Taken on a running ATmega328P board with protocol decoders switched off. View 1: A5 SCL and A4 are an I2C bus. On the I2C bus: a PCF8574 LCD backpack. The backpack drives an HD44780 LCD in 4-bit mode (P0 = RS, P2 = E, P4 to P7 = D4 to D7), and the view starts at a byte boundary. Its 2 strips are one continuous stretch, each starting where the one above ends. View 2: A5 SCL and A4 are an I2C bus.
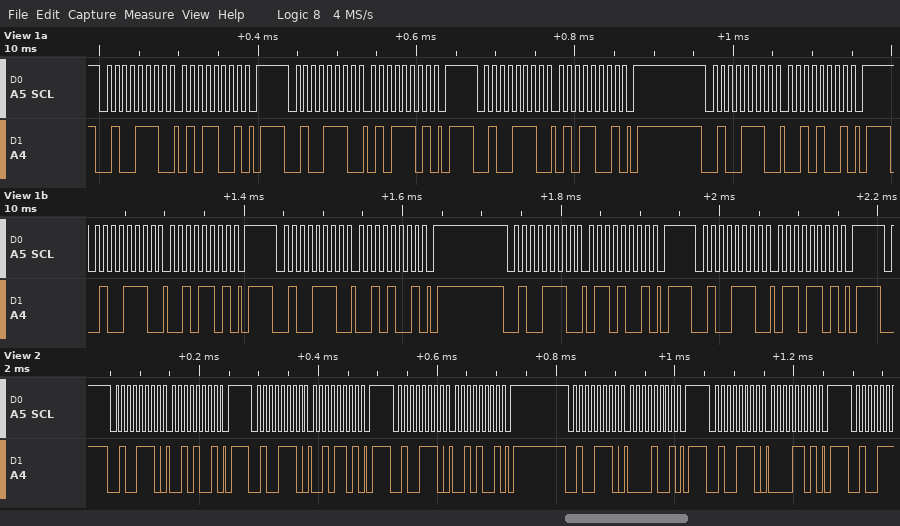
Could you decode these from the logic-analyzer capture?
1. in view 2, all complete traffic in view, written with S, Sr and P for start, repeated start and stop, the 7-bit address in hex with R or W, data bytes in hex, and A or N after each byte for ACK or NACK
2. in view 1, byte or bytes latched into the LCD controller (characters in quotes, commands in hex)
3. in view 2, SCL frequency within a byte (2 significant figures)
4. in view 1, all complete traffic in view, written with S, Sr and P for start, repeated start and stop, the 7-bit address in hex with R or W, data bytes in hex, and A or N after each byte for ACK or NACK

S 27W A 29 A P S 27W A 2D A P S 27W A 29 A P S 27W A 09 A P S 27W A 0D A P
'R'
100 kHz
S 27W A 59 A P S 27W A 5D A P S 27W A 59 A P S 27W A 29 A P S 27W A 2D A P S 27W A 29 A P S 27W A 69 A P S 27W A 6D A P
